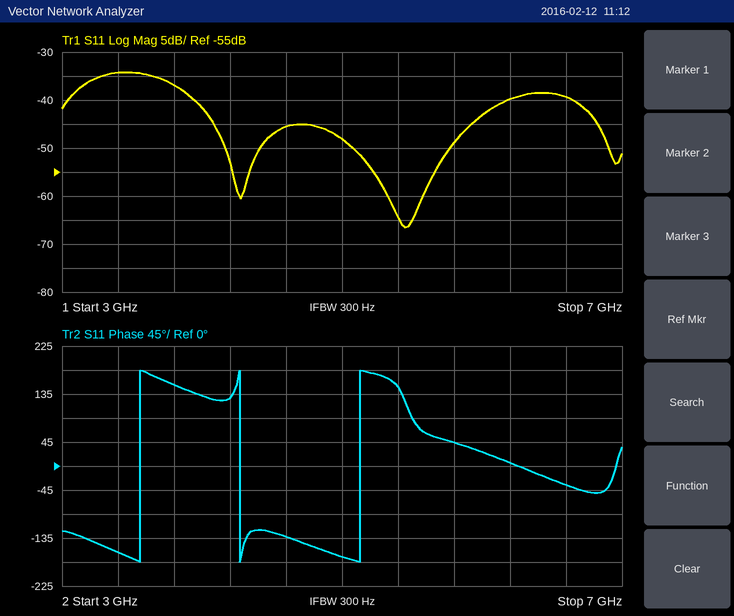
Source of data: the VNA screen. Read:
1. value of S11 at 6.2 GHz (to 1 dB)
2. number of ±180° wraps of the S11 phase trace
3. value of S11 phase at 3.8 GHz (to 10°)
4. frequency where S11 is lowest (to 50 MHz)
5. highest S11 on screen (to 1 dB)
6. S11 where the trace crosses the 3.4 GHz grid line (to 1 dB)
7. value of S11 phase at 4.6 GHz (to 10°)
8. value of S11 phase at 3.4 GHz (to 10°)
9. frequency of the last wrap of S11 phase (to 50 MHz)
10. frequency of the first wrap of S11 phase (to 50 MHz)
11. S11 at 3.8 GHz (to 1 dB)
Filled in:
-40 dB
3
150°
5.45 GHz
-34 dB
-34 dB
-130°
-160°
5.15 GHz
3.55 GHz
-37 dB
